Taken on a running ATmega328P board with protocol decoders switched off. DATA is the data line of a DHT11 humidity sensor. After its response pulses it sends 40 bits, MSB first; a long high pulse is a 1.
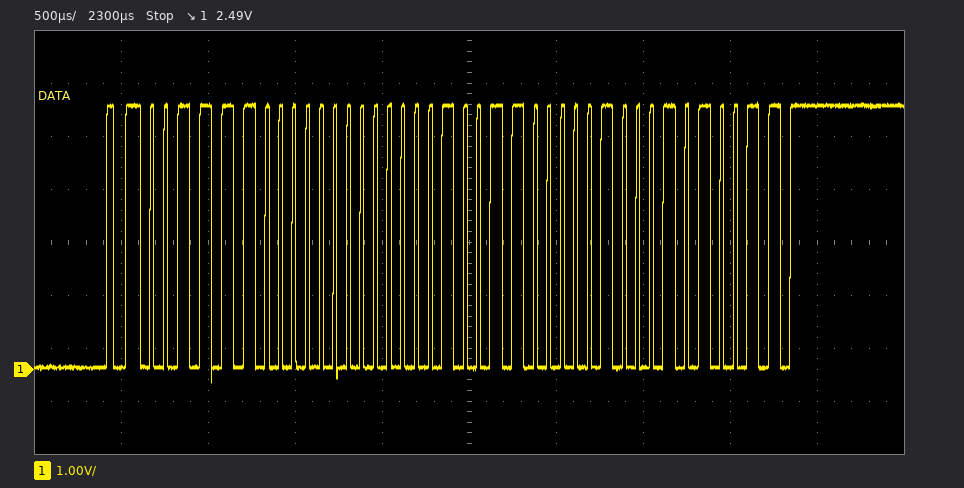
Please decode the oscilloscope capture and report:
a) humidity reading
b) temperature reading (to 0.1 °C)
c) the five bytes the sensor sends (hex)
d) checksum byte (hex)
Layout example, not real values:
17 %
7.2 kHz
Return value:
60 %
19.4 °C
3C 00 13 04 53
0x53
